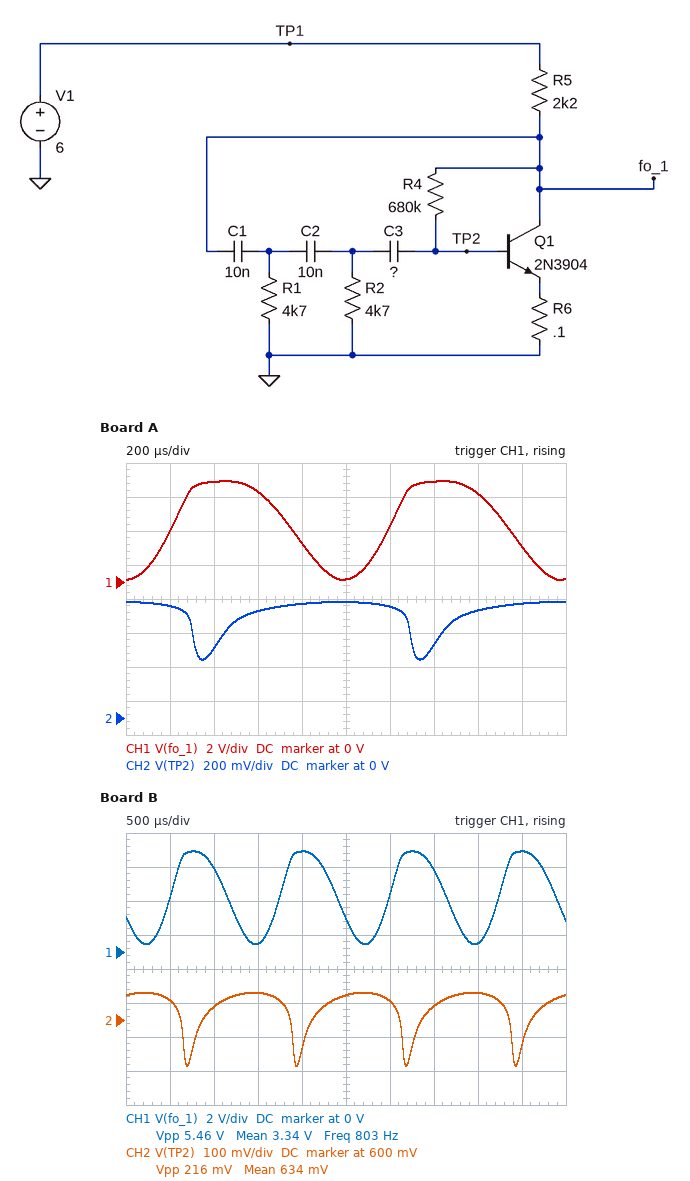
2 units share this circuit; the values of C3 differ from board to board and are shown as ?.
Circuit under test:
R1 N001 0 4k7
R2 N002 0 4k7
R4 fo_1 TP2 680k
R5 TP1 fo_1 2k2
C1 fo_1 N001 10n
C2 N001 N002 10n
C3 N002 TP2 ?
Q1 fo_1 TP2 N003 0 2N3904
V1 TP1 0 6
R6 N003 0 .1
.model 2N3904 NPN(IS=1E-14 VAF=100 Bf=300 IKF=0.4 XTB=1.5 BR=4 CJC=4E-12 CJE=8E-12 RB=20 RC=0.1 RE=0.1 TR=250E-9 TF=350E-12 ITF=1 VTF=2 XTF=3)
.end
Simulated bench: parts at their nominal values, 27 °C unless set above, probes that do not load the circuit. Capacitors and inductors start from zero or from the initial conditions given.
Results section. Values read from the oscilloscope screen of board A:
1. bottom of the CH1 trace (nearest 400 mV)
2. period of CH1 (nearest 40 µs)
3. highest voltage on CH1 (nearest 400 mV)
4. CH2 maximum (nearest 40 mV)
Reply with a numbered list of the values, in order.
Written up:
1. 0 V
2. 1.00 ms
3. 6.0 V
4. 680 mV
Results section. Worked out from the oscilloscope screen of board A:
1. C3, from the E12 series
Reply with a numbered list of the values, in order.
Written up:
1. 8.2 nF
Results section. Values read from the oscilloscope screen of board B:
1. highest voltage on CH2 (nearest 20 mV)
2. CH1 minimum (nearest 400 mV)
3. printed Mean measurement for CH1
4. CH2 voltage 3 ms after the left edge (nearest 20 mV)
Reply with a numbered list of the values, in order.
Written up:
1. 680 mV
2. 400 mV
3. 3.34 V
4. 660 mV
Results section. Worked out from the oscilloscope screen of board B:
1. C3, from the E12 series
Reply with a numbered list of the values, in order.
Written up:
1. 18 nF
